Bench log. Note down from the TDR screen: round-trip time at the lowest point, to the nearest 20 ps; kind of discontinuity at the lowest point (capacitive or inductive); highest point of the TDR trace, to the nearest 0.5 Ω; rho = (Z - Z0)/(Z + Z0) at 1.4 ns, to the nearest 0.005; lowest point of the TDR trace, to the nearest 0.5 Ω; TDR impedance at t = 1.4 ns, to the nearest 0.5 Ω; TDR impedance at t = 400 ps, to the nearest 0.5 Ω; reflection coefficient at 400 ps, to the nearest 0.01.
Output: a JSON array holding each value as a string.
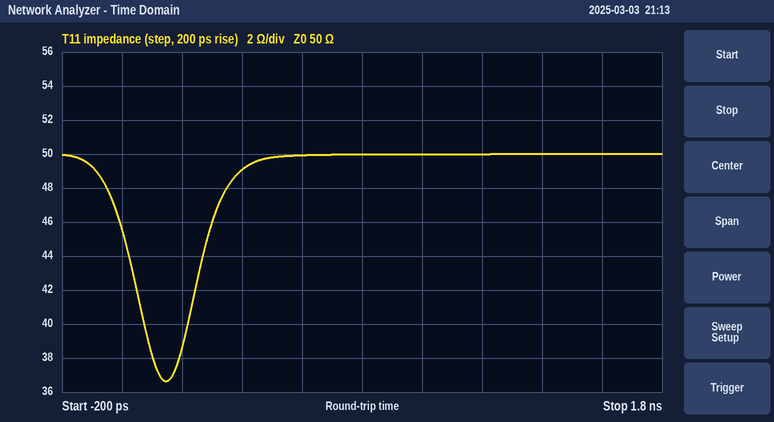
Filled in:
["140 ps", "capacitive", "50.0 Ω", "0.000", "36.5 Ω", "50.0 Ω", "49.0 Ω", "-0.01"]
